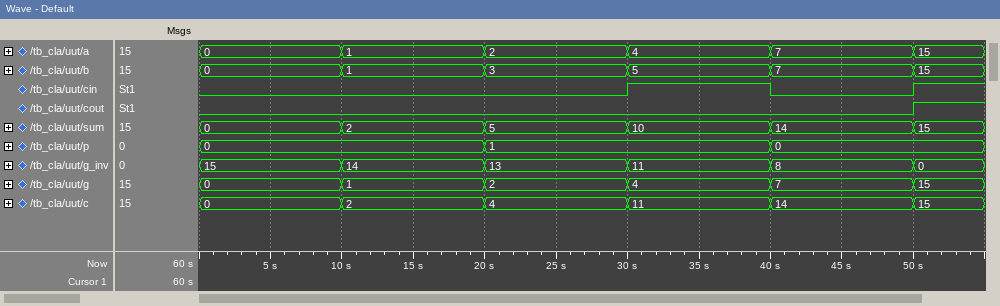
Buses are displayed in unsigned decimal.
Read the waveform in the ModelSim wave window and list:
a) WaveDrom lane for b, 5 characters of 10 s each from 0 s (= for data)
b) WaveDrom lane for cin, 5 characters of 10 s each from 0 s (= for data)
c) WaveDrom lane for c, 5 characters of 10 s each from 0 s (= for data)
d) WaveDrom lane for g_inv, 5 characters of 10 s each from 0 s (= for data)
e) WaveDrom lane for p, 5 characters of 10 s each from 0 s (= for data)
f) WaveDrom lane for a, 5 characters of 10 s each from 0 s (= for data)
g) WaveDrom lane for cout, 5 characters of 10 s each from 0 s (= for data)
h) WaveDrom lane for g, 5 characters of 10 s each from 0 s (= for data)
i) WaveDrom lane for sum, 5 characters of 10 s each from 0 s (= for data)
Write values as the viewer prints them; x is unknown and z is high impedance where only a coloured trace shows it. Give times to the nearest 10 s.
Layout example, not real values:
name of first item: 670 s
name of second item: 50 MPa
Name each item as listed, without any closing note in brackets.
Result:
WaveDrom lane for b, 5 characters of 10 s each from 0 s: {name: 'b', wave: '=====', data: '0 1 3 5 7'}
WaveDrom lane for cin, 5 characters of 10 s each from 0 s: {name: 'cin', wave: '0..10'}
WaveDrom lane for c, 5 characters of 10 s each from 0 s: {name: 'c', wave: '=====', data: '0 2 4 11 14'}
WaveDrom lane for g_inv, 5 characters of 10 s each from 0 s: {name: 'g_inv', wave: '=====', data: '15 14 13 11 8'}
WaveDrom lane for p, 5 characters of 10 s each from 0 s: {name: 'p', wave: '=.=.=', data: '0 1 0'}
WaveDrom lane for a, 5 characters of 10 s each from 0 s: {name: 'a', wave: '=====', data: '0 1 2 4 7'}
WaveDrom lane for cout, 5 characters of 10 s each from 0 s: {name: 'cout', wave: '0....'}
WaveDrom lane for g, 5 characters of 10 s each from 0 s: {name: 'g', wave: '=====', data: '0 1 2 4 7'}
WaveDrom lane for sum, 5 characters of 10 s each from 0 s: {name: 'sum', wave: '=====', data: '0 2 5 10 14'}
